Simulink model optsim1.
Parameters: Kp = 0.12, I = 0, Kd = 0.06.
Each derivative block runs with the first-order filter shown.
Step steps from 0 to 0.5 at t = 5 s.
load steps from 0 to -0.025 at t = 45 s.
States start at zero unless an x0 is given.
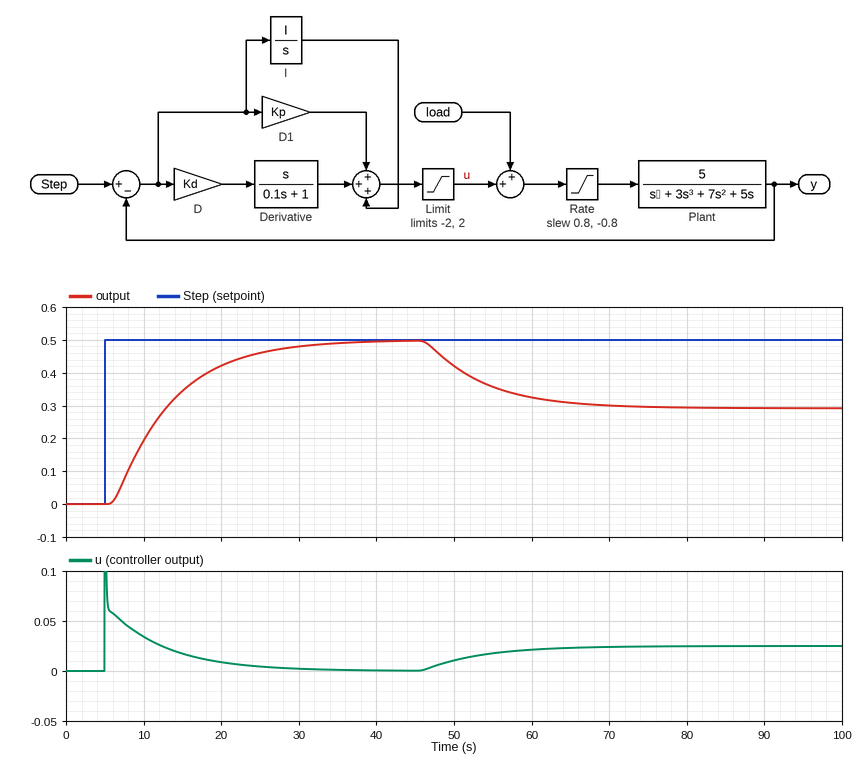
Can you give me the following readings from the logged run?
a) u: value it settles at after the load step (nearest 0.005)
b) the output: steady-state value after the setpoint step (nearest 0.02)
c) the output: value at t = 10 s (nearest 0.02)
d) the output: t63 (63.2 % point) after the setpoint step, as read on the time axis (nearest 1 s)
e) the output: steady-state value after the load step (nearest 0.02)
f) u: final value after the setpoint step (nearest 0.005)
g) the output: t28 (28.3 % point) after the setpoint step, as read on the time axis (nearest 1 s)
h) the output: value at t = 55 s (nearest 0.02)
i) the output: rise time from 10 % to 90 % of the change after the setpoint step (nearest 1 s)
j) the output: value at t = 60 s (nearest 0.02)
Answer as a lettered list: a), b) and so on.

a) 0.025
b) 0.50
c) 0.20
d) 14 s
e) 0.30
f) 0.000
g) 9 s
h) 0.36
i) 16 s
j) 0.32
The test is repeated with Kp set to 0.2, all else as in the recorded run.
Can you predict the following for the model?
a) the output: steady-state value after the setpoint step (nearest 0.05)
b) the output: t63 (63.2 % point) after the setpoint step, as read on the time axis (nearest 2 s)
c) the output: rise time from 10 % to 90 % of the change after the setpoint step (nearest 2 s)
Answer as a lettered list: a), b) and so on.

a) 0.50
b) 10 s
c) 8 s
